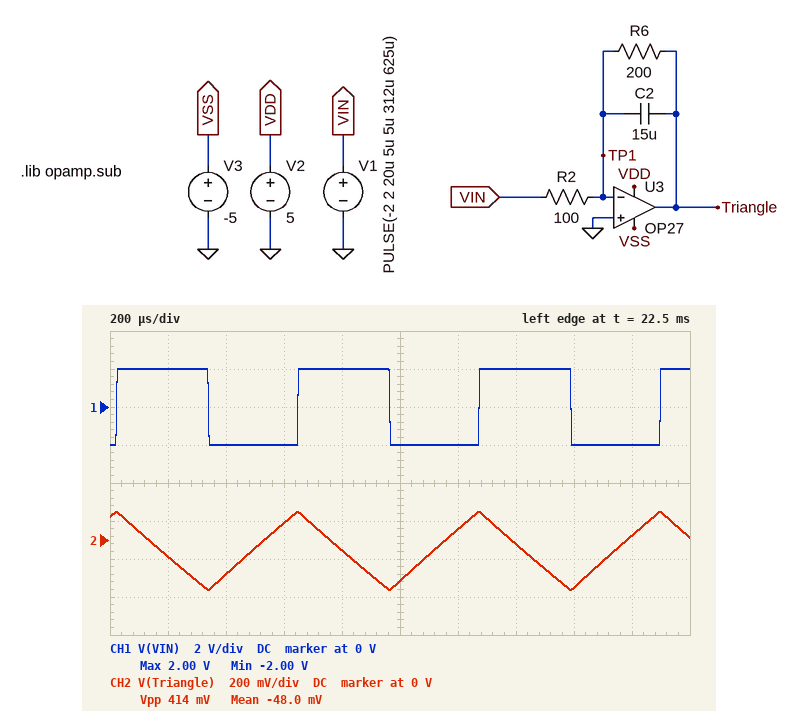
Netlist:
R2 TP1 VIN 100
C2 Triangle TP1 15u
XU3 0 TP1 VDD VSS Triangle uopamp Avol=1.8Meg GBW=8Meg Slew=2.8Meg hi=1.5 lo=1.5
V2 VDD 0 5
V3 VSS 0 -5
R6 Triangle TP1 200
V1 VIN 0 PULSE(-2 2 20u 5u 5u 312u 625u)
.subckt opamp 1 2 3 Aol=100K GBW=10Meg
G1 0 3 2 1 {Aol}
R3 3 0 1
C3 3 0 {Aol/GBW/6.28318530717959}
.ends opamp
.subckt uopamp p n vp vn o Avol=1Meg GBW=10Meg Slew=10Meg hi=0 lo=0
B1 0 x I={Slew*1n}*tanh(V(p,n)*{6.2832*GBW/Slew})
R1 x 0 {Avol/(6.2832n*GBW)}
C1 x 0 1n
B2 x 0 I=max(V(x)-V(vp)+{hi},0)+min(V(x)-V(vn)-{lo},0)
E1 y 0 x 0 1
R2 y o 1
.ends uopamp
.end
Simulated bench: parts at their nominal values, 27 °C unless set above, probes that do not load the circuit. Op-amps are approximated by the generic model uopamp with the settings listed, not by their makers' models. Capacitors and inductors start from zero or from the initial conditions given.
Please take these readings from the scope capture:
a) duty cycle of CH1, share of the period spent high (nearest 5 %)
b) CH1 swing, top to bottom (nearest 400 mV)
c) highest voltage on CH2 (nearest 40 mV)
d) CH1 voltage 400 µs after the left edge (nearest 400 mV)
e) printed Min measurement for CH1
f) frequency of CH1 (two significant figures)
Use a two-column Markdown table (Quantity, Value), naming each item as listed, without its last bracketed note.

| Quantity | Value |
|---|---|
| duty cycle of CH1, share of the period spent high | 50 % |
| CH1 swing, top to bottom | 4.0 V |
| highest voltage on CH2 | 160 mV |
| CH1 voltage 400 µs after the left edge | -2.0 V |
| printed Min measurement for CH1 | -2.00 V |
| frequency of CH1 | 1.6 kHz |
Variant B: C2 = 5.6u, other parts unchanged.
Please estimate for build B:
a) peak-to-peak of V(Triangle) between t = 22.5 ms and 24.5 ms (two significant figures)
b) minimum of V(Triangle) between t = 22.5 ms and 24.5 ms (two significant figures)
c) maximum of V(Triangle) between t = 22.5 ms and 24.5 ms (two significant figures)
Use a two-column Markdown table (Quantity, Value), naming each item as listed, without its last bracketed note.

| Quantity | Value |
|---|---|
| peak-to-peak of V(Triangle) between t = 22.5 ms and 24.5 ms | 1.1 V |
| minimum of V(Triangle) between t = 22.5 ms and 24.5 ms | -610 mV |
| maximum of V(Triangle) between t = 22.5 ms and 24.5 ms | 490 mV |
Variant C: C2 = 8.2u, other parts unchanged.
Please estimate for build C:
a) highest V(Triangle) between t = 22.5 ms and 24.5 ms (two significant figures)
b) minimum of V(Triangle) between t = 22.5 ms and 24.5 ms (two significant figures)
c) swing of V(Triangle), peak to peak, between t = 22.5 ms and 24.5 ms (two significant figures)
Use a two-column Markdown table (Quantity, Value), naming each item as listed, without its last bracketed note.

| Quantity | Value |
|---|---|
| highest V(Triangle) between t = 22.5 ms and 24.5 ms | 320 mV |
| minimum of V(Triangle) between t = 22.5 ms and 24.5 ms | -430 mV |
| swing of V(Triangle), peak to peak, between t = 22.5 ms and 24.5 ms | 750 mV |
